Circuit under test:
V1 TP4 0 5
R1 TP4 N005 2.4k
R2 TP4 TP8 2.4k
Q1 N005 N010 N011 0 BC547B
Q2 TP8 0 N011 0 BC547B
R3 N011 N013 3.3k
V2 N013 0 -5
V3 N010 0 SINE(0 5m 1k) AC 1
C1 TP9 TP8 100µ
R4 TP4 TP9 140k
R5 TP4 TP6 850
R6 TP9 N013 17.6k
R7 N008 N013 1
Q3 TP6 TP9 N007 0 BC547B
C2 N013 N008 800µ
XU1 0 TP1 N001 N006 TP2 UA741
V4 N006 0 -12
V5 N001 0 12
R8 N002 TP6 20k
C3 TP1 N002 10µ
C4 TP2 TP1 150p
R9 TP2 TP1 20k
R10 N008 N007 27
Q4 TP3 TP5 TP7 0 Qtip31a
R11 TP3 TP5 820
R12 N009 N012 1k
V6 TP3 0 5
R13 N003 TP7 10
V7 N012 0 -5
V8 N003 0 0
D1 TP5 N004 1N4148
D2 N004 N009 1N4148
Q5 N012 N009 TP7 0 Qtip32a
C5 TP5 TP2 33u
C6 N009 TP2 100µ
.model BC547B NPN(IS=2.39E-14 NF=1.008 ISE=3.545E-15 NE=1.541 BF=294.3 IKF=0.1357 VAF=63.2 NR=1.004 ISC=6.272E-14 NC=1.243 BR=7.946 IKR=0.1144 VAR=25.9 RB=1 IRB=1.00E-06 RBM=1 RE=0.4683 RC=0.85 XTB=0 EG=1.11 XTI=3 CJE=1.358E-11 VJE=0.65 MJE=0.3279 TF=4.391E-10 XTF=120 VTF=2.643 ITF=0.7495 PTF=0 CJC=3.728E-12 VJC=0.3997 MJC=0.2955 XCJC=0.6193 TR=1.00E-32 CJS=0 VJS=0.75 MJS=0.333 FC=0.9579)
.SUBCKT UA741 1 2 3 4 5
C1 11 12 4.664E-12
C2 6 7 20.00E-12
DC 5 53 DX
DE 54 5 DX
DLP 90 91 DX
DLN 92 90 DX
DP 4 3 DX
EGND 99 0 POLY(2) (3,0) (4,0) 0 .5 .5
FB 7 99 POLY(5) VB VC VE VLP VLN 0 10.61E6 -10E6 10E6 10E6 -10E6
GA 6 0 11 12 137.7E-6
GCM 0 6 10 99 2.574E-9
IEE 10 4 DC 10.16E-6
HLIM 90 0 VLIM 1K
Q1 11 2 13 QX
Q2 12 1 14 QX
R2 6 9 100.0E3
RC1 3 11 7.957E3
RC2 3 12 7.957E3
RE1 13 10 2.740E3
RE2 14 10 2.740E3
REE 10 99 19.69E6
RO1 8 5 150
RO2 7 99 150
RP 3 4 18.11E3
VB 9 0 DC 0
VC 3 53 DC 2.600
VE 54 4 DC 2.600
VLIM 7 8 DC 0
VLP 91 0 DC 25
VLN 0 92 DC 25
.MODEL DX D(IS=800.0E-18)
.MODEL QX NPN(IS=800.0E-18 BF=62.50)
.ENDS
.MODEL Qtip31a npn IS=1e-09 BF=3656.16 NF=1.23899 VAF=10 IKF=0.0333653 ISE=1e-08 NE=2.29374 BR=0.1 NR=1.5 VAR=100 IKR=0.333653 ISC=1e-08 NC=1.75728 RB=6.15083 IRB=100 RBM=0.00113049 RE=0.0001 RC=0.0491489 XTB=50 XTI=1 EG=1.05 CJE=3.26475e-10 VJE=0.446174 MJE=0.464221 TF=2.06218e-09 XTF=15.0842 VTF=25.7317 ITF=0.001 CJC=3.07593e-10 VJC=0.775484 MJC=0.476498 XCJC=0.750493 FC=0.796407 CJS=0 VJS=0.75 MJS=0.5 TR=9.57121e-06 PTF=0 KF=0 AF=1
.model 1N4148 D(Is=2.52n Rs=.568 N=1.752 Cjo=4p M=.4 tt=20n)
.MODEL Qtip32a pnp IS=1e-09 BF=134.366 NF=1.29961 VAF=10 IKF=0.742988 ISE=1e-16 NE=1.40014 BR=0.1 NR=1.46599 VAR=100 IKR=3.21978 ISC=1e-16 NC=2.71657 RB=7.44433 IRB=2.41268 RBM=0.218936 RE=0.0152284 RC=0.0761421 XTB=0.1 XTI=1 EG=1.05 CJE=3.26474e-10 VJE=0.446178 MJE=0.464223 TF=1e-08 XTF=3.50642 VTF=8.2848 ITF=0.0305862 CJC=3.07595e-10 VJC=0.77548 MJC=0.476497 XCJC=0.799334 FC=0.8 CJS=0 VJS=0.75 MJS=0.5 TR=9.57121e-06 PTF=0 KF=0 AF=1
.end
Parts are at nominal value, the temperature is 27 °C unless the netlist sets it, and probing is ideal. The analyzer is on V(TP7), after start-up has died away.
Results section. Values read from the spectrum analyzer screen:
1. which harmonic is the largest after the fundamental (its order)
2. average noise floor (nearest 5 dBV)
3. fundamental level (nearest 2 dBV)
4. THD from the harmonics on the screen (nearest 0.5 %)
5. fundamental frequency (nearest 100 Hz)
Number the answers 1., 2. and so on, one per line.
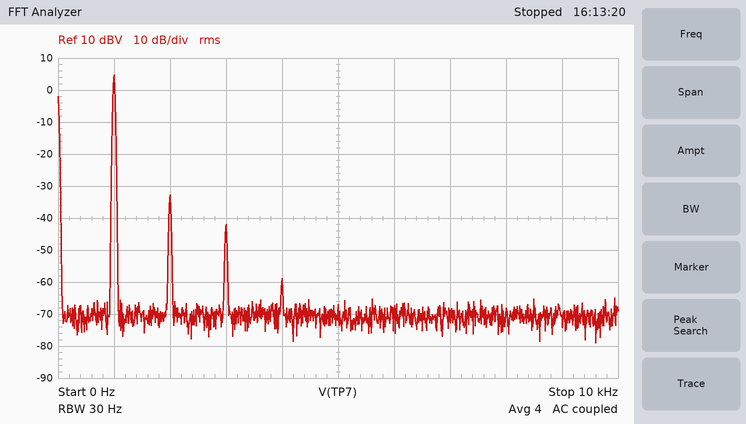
1. 2
2. -70 dBV
3. 4 dBV
4. 1.5 %
5. 1.0 kHz
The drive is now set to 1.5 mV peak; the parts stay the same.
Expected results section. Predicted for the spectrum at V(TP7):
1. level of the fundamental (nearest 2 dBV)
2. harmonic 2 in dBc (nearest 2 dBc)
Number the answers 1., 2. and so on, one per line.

1. -6 dBV
2. -50 dBc
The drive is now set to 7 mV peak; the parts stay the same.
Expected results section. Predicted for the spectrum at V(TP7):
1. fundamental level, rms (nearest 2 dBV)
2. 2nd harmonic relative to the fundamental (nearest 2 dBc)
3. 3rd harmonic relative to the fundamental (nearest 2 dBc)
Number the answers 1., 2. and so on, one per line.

1. 8 dBV
2. -32 dBc
3. -40 dBc
